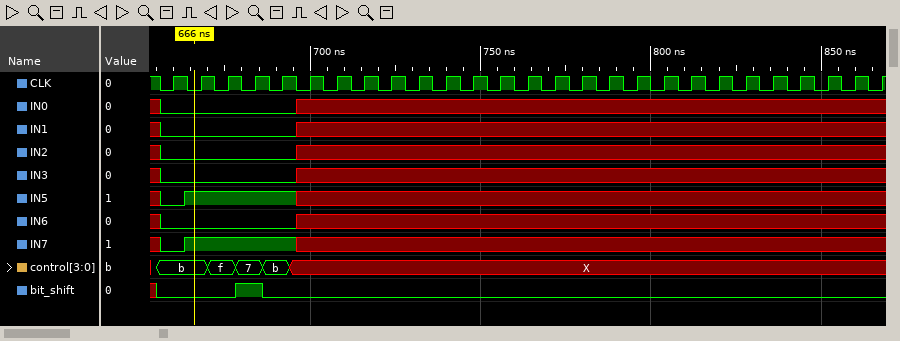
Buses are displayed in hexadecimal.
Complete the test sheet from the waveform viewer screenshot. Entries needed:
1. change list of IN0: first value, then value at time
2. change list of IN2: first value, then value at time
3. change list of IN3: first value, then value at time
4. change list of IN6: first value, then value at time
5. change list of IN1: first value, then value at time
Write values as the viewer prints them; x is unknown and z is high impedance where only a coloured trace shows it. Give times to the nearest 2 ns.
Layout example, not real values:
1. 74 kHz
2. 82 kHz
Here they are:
1. x, 0 at 656 ns, x at 696 ns
2. x, 0 at 656 ns, x at 696 ns
3. x, 0 at 656 ns, x at 696 ns
4. x, 0 at 656 ns, x at 696 ns
5. x, 0 at 656 ns, x at 696 ns
